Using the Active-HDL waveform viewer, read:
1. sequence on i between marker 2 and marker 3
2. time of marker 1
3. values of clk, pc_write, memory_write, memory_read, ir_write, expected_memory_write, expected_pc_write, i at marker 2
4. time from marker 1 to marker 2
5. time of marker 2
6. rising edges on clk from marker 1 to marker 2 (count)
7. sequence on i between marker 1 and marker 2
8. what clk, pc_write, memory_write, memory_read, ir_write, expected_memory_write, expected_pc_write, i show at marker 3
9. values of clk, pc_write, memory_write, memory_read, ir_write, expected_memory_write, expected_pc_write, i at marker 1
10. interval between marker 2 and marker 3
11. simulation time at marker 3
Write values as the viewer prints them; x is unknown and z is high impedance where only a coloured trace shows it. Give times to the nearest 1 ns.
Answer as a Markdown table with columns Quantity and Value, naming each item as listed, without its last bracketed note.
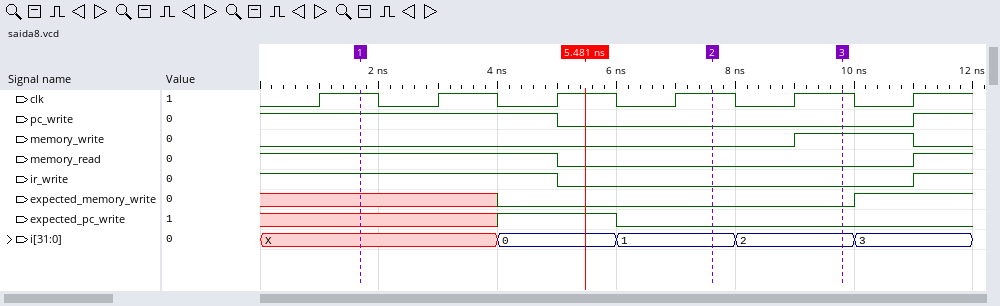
| Quantity | Value |
|---|---|
| sequence on i between marker 2 and marker 3 | 1, 2 |
| time of marker 1 | 2 ns |
| values of clk, pc_write, memory_write, memory_read, ir_write, expected_memory_write, expected_pc_write, i at marker 2 | clk=1, pc_write=0, memory_write=0, memory_read=0, ir_write=0, expected_memory_write=0, expected_pc_write=0, i=1 |
| time from marker 1 to marker 2 | 6 ns |
| time of marker 2 | 8 ns |
| rising edges on clk from marker 1 to marker 2 | 3 |
| sequence on i between marker 1 and marker 2 | X, 0, 1 |
| what clk, pc_write, memory_write, memory_read, ir_write, expected_memory_write, expected_pc_write, i show at marker 3 | clk=1, pc_write=0, memory_write=1, memory_read=0, ir_write=0, expected_memory_write=0, expected_pc_write=0, i=2 |
| values of clk, pc_write, memory_write, memory_read, ir_write, expected_memory_write, expected_pc_write, i at marker 1 | clk=1, pc_write=1, memory_write=0, memory_read=1, ir_write=1, expected_memory_write=x, expected_pc_write=x, i=X |
| interval between marker 2 and marker 3 | 2 ns |
| simulation time at marker 3 | 10 ns |
